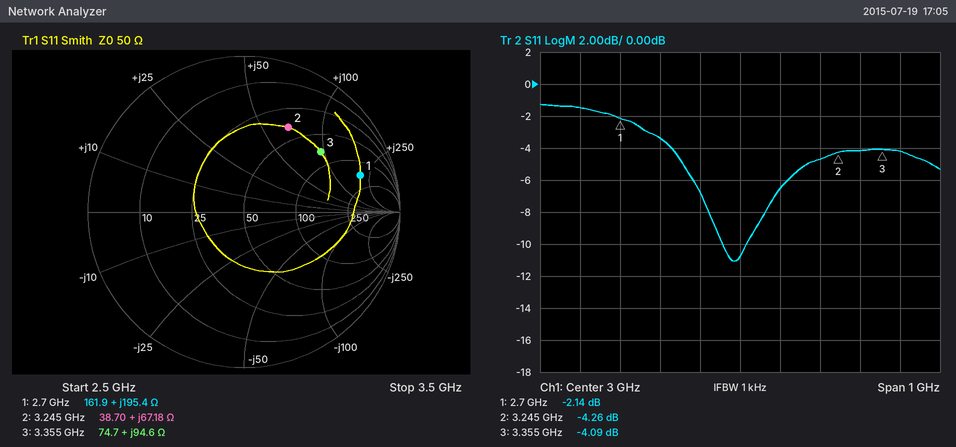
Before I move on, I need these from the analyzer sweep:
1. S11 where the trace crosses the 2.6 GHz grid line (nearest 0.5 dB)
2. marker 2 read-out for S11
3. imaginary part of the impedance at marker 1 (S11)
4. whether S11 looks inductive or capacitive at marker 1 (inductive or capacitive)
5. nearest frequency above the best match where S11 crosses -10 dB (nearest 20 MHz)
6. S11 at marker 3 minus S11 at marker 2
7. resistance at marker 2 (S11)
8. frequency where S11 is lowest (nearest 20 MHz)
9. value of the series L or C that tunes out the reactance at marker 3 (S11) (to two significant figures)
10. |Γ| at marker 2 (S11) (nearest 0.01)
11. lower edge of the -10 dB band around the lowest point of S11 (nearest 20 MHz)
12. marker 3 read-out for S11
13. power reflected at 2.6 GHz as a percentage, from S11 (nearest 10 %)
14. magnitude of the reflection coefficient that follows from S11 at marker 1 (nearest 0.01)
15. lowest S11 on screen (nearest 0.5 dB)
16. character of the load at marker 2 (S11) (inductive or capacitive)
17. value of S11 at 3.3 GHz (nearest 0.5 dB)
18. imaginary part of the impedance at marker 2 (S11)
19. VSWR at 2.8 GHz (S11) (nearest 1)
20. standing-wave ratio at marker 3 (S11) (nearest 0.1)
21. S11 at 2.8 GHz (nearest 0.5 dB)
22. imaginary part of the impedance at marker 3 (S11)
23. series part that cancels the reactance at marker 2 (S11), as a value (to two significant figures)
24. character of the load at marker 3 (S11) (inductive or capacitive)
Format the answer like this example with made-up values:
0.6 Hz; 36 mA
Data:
-1.5 dB; -4.26 dB; +195.4 Ω; inductive; 3.02 GHz; 0.17 dB; 38.70 Ω; 2.98 GHz; 500 fF; 0.61; 2.96 GHz; -4.09 dB; 70 %; 0.78; -11.0 dB; inductive; -4.0 dB; +67.18 Ω; 5; 4.3; -3.5 dB; +94.6 Ω; 730 fF; inductive
